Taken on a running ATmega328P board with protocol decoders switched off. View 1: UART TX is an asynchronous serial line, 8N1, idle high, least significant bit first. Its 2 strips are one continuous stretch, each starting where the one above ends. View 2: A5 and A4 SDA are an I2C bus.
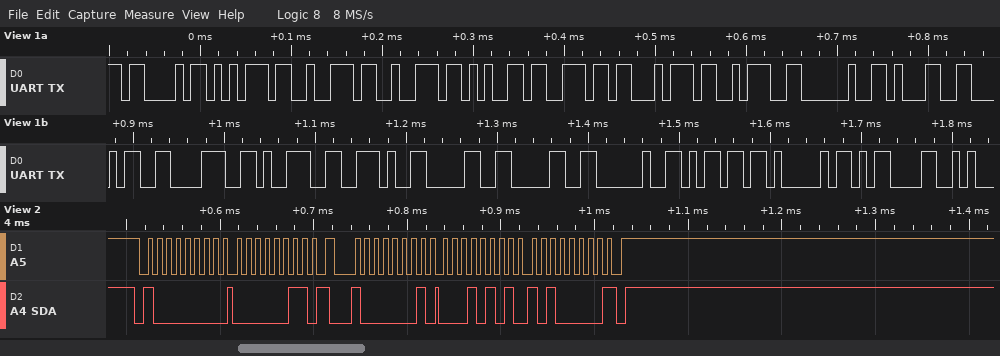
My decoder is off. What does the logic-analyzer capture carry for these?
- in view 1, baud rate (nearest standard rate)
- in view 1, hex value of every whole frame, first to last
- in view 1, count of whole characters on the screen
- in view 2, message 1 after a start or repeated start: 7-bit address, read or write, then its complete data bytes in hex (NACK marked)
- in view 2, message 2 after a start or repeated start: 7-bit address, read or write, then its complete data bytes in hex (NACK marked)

115200 baud
43 75 72 72 65 6E 74 3A 20 31 34 38 39 2E 30 30 20 6D 41 0D
20
0x40 write: 03
0x40 read: 15 A0 NACK
